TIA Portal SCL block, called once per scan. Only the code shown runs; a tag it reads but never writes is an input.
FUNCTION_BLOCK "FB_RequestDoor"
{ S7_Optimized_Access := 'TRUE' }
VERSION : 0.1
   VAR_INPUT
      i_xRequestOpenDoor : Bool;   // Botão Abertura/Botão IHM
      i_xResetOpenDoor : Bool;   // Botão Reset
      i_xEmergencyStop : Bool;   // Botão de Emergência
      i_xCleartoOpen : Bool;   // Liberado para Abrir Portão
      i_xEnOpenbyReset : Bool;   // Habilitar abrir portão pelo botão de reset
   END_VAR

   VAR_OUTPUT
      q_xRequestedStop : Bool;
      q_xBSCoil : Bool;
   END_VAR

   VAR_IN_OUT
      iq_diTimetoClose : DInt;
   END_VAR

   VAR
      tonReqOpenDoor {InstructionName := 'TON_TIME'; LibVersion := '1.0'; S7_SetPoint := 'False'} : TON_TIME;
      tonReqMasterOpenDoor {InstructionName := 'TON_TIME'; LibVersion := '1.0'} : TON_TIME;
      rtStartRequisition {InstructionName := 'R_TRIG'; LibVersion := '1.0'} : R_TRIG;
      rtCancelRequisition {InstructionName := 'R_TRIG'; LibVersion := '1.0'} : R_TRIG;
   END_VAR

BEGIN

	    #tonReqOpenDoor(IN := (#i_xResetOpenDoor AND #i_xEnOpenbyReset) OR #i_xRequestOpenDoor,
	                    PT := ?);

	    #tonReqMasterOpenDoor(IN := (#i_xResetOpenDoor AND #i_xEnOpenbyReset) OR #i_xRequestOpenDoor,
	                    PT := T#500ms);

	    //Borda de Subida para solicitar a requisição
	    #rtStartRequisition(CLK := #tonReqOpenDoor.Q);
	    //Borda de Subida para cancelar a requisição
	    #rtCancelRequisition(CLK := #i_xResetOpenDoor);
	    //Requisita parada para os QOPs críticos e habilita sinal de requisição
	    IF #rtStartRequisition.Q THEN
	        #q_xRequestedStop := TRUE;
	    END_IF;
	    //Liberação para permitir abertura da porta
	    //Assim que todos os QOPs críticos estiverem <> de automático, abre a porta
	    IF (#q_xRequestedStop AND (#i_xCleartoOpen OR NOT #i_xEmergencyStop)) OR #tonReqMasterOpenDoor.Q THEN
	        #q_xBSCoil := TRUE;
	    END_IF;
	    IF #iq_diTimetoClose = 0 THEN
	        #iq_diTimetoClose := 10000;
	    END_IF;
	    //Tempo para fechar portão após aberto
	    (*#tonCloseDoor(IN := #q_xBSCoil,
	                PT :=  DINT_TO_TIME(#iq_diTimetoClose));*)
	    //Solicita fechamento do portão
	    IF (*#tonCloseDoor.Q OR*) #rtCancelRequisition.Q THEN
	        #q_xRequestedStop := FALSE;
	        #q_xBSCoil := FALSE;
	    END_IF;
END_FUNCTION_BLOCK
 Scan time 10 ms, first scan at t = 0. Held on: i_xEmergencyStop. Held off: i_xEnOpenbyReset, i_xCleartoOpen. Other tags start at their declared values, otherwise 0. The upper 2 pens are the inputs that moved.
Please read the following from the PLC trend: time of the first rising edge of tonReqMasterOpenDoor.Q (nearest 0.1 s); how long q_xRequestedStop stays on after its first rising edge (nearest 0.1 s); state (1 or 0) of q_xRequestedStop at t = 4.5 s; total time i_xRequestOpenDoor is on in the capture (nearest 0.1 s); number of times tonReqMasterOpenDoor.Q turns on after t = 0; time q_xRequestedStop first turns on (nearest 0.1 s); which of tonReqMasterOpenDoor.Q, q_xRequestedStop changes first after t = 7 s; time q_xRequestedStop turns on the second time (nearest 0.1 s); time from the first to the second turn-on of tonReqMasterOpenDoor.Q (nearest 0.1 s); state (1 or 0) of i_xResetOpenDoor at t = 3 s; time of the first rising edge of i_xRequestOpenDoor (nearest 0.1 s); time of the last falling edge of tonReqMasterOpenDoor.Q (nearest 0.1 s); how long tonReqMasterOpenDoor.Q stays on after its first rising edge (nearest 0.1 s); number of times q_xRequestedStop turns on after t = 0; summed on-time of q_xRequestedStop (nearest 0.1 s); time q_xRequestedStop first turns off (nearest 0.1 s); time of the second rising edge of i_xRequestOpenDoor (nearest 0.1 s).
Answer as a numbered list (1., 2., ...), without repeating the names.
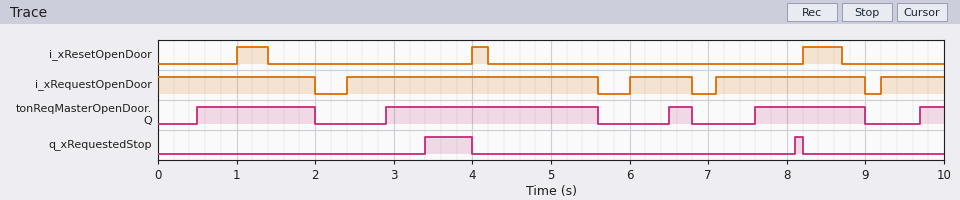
1. 0.5 s
2. 0.6 s
3. 0
4. 8.7 s
5. 5
6. 3.4 s
7. tonReqMasterOpenDoor.Q
8. 8.1 s
9. 2.4 s
10. 0
11. 2.4 s
12. 9.0 s
13. 1.5 s
14. 2
15. 0.7 s
16. 4.0 s
17. 6.0 s
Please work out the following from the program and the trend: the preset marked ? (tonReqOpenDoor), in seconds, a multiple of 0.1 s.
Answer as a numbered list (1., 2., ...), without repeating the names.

1. 1.0 s
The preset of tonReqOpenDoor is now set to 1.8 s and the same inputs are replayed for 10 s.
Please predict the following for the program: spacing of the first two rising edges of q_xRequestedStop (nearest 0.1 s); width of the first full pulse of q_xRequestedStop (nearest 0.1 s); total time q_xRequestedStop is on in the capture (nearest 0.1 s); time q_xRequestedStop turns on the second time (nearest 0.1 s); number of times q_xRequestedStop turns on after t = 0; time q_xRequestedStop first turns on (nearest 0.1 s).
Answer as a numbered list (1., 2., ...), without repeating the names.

1. 2.4 s
2. 2.2 s
3. 7.3 s
4. 4.2 s
5. 3
6. 1.8 s
